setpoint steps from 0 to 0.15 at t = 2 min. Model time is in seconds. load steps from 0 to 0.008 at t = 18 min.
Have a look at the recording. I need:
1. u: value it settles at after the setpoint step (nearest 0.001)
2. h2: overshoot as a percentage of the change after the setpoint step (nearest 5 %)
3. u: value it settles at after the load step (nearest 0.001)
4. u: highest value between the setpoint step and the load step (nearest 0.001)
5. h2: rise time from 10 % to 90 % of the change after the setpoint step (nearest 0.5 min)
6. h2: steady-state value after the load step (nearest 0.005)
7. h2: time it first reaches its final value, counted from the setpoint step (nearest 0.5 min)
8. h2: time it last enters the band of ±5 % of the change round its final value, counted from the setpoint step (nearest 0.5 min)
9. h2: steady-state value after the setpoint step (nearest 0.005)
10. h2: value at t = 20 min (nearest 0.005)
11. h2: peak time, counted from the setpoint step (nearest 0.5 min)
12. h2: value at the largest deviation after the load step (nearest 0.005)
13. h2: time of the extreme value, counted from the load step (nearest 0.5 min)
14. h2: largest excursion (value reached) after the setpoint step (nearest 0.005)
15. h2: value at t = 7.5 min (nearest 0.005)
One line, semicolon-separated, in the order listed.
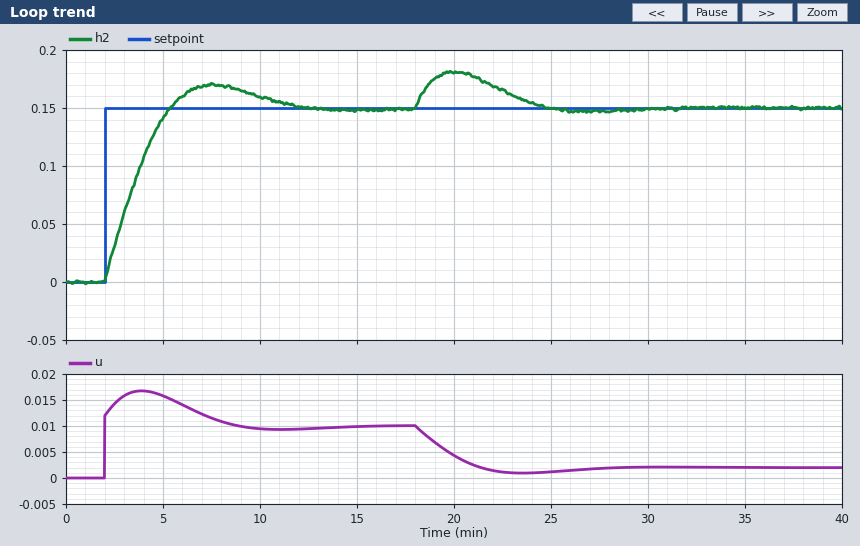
0.010; 15 %; 0.002; 0.017; 2.5 min; 0.150; 3.5 min; 8.5 min; 0.150; 0.180; 5.5 min; 0.180; 2.0 min; 0.170; 0.170
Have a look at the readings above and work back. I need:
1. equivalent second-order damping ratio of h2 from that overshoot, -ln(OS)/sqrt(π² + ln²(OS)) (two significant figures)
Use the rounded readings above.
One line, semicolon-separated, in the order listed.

0.52
